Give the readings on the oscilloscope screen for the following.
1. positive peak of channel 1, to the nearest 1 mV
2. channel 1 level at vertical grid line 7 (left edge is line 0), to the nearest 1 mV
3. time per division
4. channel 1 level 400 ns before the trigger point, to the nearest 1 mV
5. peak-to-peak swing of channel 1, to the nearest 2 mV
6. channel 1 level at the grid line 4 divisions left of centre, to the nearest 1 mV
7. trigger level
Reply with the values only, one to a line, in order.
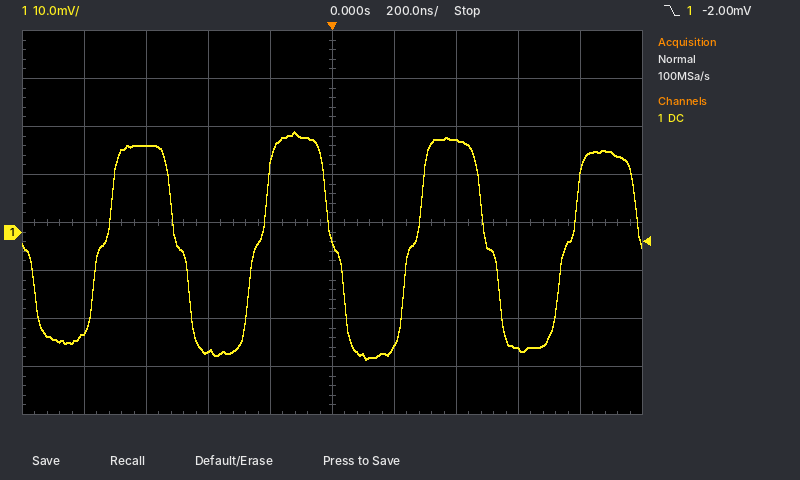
21 mV
19 mV
200 ns
-25 mV
48 mV
-21 mV
-2.00 mV
